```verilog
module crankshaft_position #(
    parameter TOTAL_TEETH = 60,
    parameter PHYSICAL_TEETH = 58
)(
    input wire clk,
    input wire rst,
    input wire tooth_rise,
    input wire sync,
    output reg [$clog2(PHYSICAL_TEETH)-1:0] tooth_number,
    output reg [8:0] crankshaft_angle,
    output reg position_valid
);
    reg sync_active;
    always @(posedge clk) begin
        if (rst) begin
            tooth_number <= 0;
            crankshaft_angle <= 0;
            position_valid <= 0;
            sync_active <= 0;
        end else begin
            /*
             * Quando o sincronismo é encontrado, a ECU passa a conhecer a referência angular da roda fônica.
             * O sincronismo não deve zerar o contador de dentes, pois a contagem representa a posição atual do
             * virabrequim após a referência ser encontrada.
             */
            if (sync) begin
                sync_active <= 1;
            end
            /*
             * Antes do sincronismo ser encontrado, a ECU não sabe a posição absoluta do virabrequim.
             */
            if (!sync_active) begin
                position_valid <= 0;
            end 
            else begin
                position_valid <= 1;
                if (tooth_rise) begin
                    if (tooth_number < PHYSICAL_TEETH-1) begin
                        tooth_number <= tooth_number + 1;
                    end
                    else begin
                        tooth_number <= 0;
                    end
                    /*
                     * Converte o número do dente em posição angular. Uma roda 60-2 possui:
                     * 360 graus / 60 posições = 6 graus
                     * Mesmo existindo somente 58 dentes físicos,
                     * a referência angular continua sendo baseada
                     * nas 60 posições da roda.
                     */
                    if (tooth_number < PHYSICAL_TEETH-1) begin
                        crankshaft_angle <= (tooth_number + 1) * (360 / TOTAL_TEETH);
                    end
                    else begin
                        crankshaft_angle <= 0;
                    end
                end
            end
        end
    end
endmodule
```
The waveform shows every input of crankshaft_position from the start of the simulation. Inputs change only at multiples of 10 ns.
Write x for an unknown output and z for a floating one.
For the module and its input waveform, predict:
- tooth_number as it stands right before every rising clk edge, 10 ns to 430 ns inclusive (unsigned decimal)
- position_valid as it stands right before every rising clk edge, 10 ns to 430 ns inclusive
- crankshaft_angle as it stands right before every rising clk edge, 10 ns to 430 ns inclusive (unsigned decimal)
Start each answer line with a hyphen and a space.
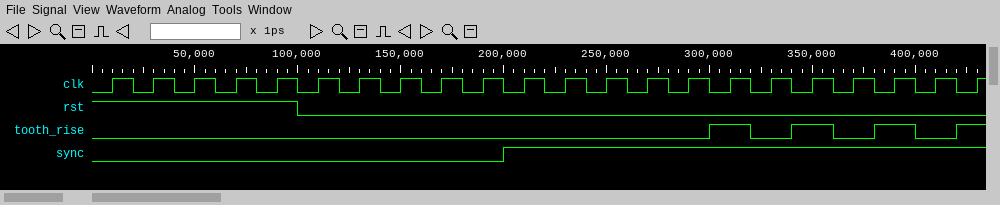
- x, 0, 0, 0, 0, 0, 0, 0, 0, 0, 0, 0, 0, 0, 0, 0, 1, 1, 2, 2, 3, 3
- x 0 0 0 0 0 0 0 0 0 0 0 1 1 1 1 1 1 1 1 1 1
- x, 0, 0, 0, 0, 0, 0, 0, 0, 0, 0, 0, 0, 0, 0, 0, 6, 6, 12, 12, 18, 18
